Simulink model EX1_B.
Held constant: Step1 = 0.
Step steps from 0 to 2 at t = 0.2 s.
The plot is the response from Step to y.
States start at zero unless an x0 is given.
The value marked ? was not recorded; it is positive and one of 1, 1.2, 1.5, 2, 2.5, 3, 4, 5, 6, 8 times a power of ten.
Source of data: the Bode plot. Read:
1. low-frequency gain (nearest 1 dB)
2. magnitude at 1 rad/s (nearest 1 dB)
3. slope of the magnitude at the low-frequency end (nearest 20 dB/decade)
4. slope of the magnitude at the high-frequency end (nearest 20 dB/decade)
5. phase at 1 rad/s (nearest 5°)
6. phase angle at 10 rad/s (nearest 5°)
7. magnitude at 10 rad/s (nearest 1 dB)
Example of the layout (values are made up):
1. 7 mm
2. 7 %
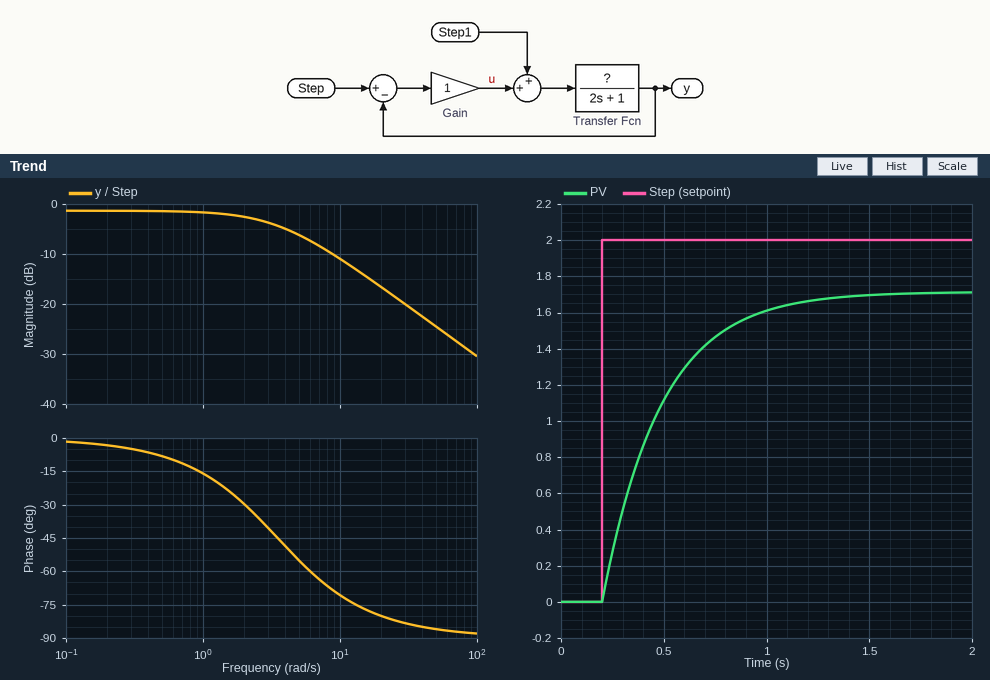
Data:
1. -1 dB
2. -2 dB
3. 0 dB/decade
4. -20 dB/decade
5. -15°
6. -70°
7. -11 dB
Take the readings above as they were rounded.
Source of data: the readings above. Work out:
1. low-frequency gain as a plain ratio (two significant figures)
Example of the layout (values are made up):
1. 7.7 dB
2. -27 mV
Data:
1. 0.89
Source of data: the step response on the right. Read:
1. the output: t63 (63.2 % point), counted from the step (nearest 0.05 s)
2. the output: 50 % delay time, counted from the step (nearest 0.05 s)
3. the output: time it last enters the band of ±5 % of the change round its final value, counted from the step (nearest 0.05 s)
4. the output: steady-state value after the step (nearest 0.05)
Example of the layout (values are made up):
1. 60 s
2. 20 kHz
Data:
1. 0.30 s
2. 0.20 s
3. 0.85 s
4. 1.70
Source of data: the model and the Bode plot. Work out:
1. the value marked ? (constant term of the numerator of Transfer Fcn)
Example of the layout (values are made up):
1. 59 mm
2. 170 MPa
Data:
1. 6
